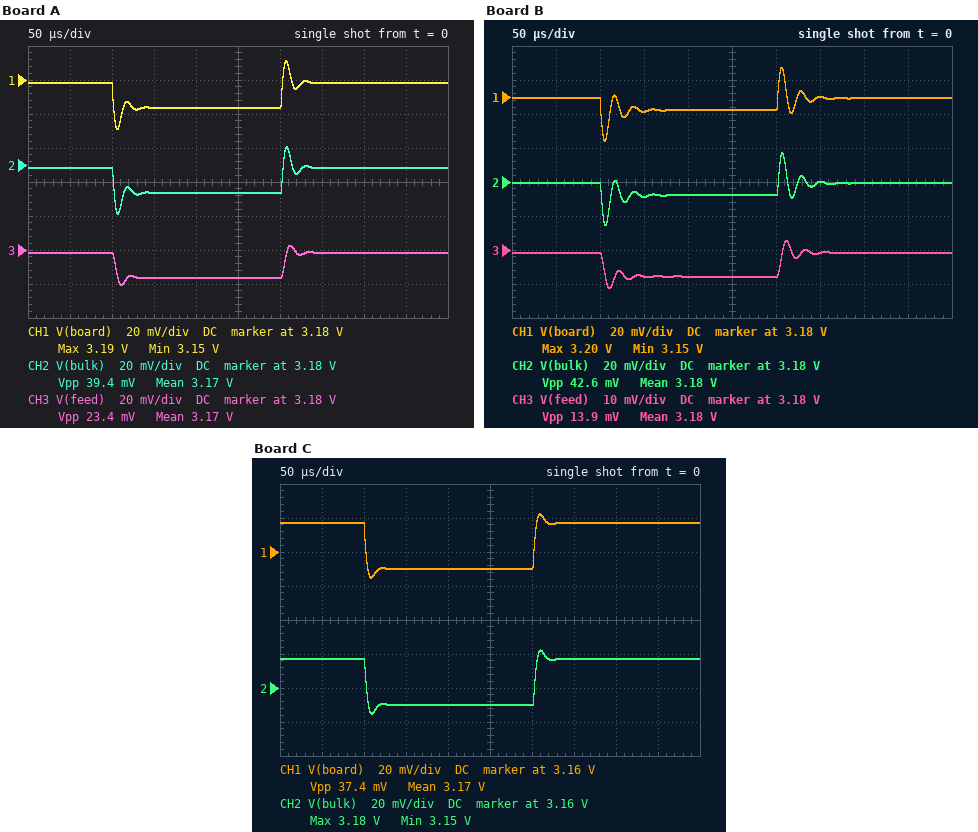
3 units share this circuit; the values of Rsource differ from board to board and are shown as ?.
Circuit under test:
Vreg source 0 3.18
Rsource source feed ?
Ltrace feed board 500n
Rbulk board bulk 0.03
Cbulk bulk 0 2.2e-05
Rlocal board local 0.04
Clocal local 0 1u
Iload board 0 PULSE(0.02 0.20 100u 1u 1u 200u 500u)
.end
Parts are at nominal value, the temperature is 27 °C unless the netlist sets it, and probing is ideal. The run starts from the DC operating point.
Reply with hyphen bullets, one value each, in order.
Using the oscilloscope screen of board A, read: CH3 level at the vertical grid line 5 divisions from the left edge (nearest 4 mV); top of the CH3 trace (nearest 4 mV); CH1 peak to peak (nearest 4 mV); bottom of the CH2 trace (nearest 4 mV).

- 3.164 V
- 3.184 V
- 40 mV
- 3.152 V
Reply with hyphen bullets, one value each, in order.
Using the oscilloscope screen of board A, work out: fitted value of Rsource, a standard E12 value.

- 0.082 Ω
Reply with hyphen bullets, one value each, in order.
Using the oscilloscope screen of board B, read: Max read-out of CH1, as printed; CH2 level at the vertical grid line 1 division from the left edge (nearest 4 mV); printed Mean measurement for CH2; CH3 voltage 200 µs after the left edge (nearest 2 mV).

- 3.20 V
- 3.180 V
- 3.18 V
- 3.172 V
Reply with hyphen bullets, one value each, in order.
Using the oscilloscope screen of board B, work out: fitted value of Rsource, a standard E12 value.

- 0.039 Ω
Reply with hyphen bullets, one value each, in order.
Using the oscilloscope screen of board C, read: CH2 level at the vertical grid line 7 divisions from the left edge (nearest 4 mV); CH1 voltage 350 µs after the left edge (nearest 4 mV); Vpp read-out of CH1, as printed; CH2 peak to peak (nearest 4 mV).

- 3.176 V
- 3.176 V
- 37.4 mV
- 36 mV
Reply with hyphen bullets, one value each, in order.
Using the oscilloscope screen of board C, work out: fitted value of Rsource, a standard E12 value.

- 0.15 Ω
